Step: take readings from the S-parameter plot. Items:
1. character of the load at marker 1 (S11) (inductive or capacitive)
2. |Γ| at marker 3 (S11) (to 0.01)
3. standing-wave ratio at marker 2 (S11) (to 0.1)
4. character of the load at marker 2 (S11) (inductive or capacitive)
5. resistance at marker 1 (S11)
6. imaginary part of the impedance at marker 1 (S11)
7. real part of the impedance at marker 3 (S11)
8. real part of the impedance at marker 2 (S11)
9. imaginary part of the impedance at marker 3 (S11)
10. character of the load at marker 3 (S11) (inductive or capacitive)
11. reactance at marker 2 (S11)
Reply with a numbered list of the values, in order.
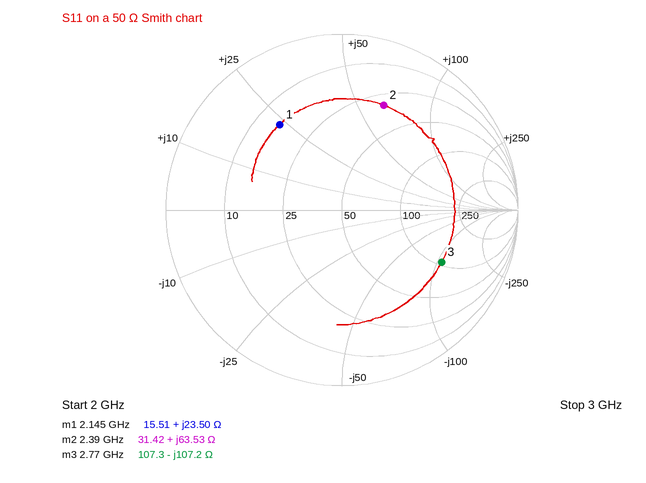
1. inductive
2. 0.64
3. 4.6
4. inductive
5. 15.51 Ω
6. +23.50 Ω
7. 107.3 Ω
8. 31.42 Ω
9. -107.2 Ω
10. capacitive
11. +63.53 Ω
